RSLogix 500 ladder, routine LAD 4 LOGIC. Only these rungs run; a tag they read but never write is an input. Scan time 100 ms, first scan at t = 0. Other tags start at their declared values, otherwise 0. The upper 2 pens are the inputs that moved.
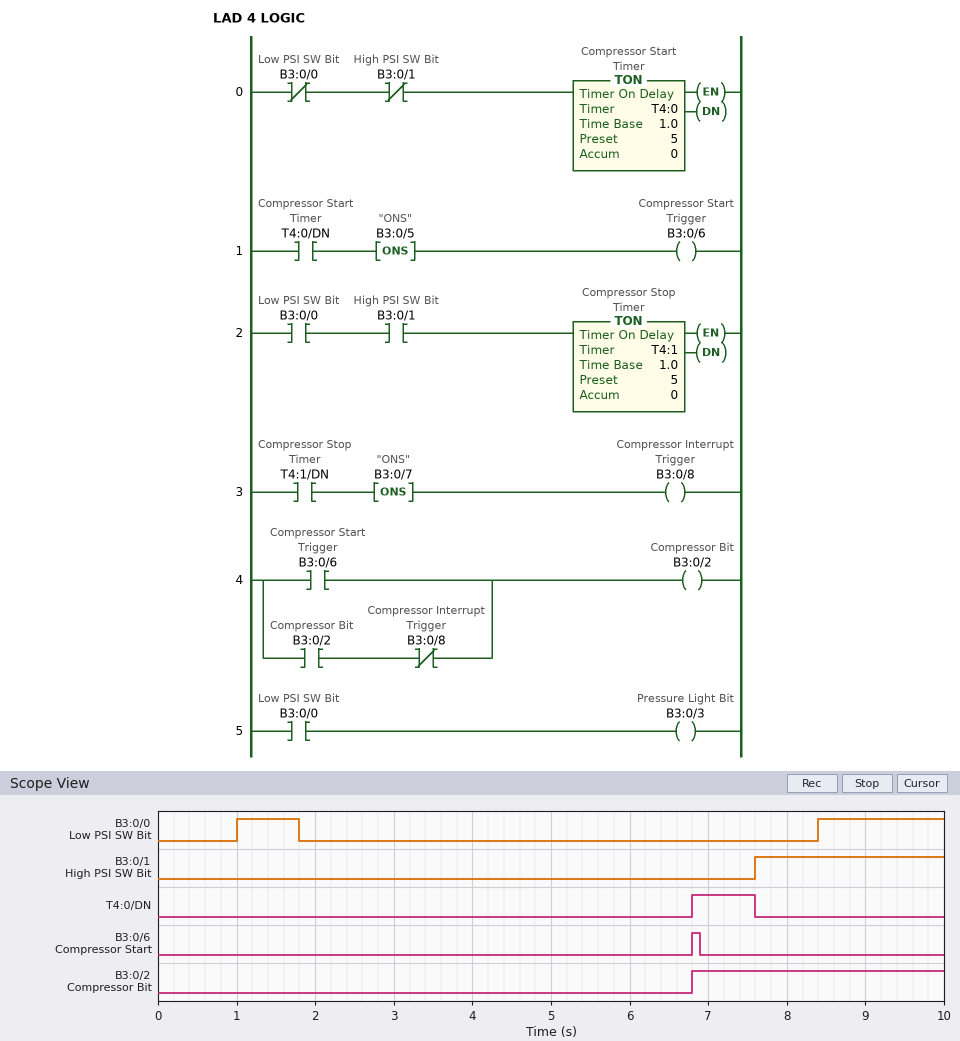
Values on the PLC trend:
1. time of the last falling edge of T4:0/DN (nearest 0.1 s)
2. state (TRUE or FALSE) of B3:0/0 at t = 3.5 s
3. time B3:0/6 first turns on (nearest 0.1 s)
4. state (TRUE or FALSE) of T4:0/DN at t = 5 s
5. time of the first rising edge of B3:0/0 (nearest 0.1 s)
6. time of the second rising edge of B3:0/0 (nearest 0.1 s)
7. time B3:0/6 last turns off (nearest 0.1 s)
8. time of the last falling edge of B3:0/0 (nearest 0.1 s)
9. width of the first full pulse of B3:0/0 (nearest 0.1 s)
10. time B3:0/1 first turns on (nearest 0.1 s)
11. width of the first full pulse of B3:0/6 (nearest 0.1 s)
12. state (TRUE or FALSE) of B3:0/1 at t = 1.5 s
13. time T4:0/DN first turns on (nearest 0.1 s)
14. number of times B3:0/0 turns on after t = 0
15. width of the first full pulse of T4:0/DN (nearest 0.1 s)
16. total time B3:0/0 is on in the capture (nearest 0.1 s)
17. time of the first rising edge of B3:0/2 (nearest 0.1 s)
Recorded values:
7.6 s
FALSE
6.8 s
FALSE
1.0 s
8.4 s
6.9 s
1.8 s
0.8 s
7.6 s
0.1 s
FALSE
6.8 s
2
0.8 s
2.4 s
6.8 s
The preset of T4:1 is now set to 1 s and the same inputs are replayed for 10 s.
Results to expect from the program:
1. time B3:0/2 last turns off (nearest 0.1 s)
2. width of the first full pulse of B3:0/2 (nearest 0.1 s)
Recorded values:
9.4 s
2.6 s
